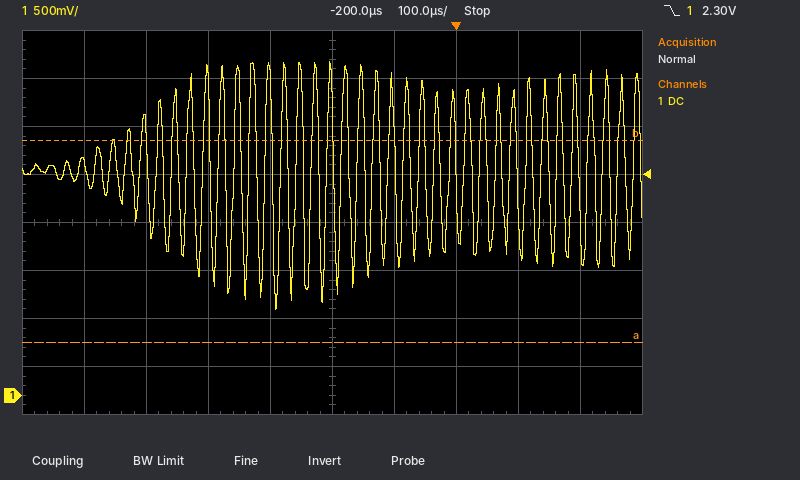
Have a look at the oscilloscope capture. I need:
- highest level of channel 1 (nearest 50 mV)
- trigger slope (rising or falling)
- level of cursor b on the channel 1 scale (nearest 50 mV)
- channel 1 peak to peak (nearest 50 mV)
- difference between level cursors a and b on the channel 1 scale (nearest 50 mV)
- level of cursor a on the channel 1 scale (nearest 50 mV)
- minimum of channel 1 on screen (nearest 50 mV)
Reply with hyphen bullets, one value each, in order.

- 3.50 V
- falling
- 2.65 V
- 2.60 V
- 2.10 V
- 550 mV
- 900 mV
